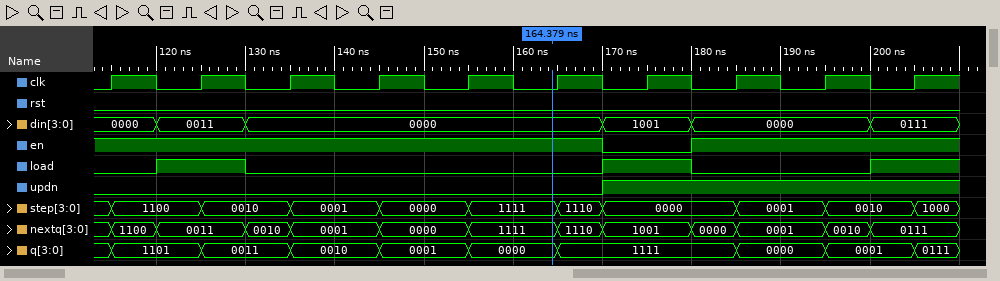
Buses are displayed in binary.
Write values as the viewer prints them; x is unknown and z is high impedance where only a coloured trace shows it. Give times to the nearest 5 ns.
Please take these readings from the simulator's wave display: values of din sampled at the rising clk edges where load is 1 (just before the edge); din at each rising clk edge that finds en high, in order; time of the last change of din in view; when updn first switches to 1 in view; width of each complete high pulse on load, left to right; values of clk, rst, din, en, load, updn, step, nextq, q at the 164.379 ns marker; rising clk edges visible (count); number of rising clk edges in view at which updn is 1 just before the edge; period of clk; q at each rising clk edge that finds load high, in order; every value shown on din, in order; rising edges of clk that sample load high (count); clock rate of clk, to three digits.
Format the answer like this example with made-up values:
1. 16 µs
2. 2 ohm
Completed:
1. 0011, 1001, 0111
2. 0000, 0011, 0000, 0000, 0000, 0000, 0000, 0000, 0111
3. 200 ns
4. 170 ns
5. 10 ns, 10 ns
6. clk=0, rst=0, din=0000, en=1, load=0, updn=0, step=1111, nextq=1111, q=0000
7. 10
8. 4
9. 10 ns
10. 1101, 1111, 0001
11. 0000, 0011, 0000, 1001, 0000, 0111
12. 3
13. 100 MHz
